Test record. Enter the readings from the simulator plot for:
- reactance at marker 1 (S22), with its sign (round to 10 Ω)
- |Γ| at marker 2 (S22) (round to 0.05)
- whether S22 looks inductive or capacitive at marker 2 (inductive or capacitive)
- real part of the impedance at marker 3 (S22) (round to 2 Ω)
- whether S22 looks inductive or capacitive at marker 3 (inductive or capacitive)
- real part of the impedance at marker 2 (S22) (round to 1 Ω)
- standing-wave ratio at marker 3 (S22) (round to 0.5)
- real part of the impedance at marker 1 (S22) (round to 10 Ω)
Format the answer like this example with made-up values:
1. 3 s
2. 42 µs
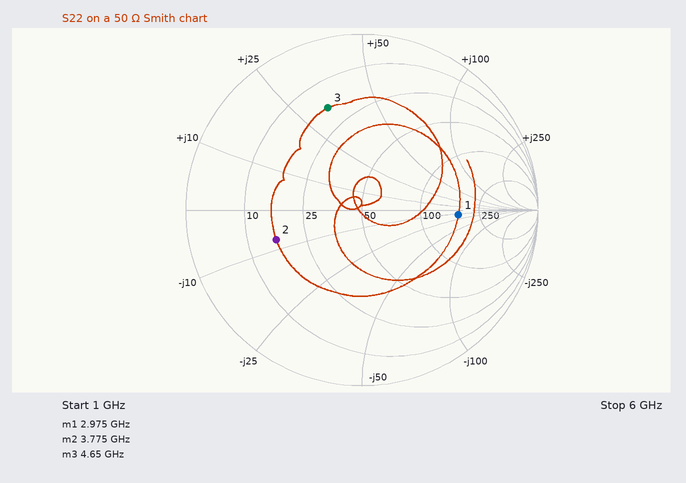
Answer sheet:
1. -10 Ω
2. 0.50
3. capacitive
4. 18 Ω
5. inductive
6. 16 Ω
7. 4.0
8. 170 Ω
